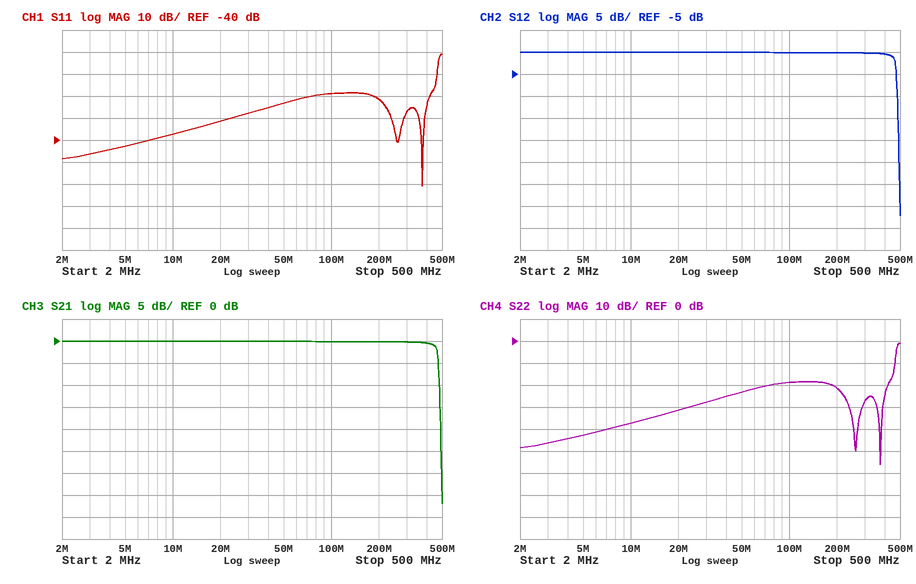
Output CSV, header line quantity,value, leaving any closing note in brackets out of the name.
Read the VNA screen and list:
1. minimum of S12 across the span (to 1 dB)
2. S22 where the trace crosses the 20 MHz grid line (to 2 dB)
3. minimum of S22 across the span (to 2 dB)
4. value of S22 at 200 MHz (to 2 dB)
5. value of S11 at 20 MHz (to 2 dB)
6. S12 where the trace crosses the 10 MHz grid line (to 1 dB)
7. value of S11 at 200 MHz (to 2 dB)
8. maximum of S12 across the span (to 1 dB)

quantity,value
minimum of S12 across the span,-37 dB
S22 where the trace crosses the 20 MHz grid line,-32 dB
minimum of S22 across the span,-56 dB
value of S22 at 200 MHz,-22 dB
value of S11 at 20 MHz,-32 dB
S12 where the trace crosses the 10 MHz grid line,0 dB
value of S11 at 200 MHz,-22 dB
maximum of S12 across the span,0 dB
